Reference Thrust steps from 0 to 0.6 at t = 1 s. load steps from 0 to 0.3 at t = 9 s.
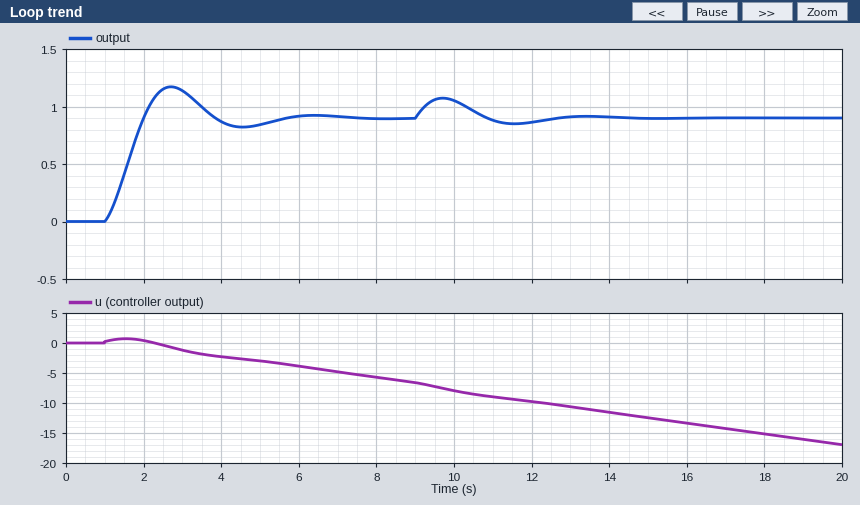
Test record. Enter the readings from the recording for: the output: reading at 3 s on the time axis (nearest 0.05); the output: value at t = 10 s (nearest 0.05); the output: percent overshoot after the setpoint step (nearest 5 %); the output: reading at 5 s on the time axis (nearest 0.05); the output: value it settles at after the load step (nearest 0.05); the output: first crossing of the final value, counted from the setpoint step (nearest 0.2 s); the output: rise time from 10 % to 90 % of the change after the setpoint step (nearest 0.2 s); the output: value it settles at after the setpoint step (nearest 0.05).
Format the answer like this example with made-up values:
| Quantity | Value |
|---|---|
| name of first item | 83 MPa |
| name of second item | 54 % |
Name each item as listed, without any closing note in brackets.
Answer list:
| Quantity | Value |
|---|---|
| the output: reading at 3 s on the time axis | 1.15 |
| the output: value at t = 10 s | 1.05 |
| the output: percent overshoot after the setpoint step | 30 % |
| the output: reading at 5 s on the time axis | 0.85 |
| the output: value it settles at after the load step | 0.90 |
| the output: first crossing of the final value, counted from the setpoint step | 1.0 s |
| the output: rise time from 10 % to 90 % of the change after the setpoint step | 0.8 s |
| the output: value it settles at after the setpoint step | 0.90 |
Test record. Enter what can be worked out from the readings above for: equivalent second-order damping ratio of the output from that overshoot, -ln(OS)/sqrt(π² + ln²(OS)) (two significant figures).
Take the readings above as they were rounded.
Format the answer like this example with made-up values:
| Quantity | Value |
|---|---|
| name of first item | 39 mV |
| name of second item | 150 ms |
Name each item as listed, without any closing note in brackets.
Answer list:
| Quantity | Value |
|---|---|
| equivalent second-order damping ratio of the output from that overshoot, -ln(OS)/sqrt(π² + ln²(OS)) | 0.36 |
